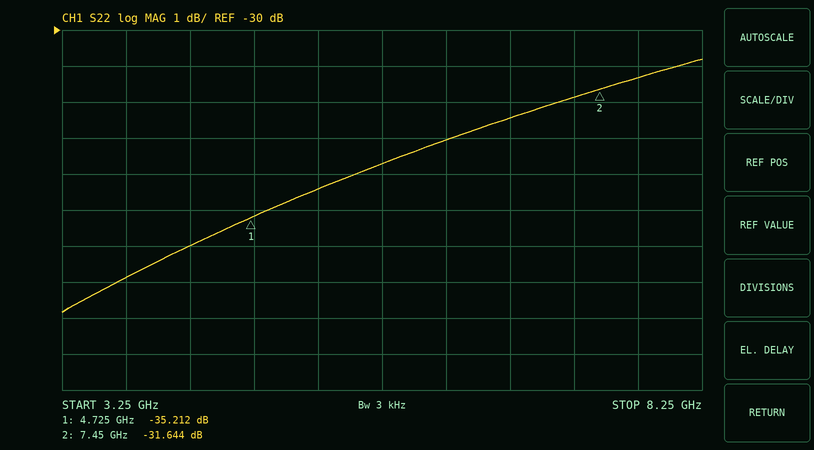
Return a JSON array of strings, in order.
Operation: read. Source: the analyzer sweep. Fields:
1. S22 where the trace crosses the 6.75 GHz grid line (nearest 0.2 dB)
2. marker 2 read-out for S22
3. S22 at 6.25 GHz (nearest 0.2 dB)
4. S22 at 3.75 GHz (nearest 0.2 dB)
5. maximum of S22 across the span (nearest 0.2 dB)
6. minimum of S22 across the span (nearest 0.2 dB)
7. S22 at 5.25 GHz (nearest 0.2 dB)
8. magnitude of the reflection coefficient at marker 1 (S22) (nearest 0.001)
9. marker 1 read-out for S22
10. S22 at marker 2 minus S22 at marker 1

["-32.4 dB", "-31.644 dB", "-33.0 dB", "-36.8 dB", "-30.8 dB", "-37.8 dB", "-34.4 dB", "0.017", "-35.212 dB", "3.568 dB"]
